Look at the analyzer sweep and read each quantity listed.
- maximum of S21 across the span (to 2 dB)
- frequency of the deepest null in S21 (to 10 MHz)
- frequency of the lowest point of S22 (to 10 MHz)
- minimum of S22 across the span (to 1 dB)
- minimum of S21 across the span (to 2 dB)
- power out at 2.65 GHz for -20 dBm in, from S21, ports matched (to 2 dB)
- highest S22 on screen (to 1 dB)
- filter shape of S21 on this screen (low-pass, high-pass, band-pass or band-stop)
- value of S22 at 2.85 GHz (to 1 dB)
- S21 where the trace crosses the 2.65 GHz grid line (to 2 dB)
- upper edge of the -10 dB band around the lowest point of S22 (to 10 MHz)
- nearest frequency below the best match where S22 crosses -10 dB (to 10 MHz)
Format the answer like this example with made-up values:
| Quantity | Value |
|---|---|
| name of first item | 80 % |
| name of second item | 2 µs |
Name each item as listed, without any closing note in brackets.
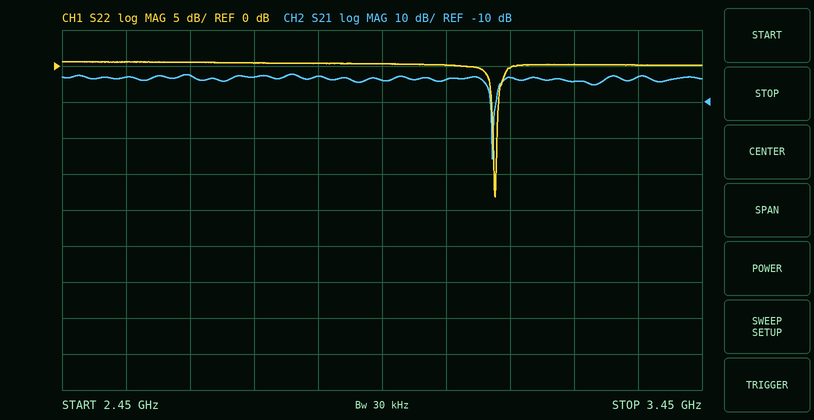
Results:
| Quantity | Value |
|---|---|
| maximum of S21 across the span | -2 dB |
| frequency of the deepest null in S21 | 3.12 GHz |
| frequency of the lowest point of S22 | 3.13 GHz |
| minimum of S22 across the span | -18 dB |
| minimum of S21 across the span | -26 dB |
| power out at 2.65 GHz for -20 dBm in, from S21, ports matched | -22 dBm |
| highest S22 on screen | 1 dB |
| filter shape of S21 on this screen | band-stop |
| value of S22 at 2.85 GHz | 0 dB |
| S21 where the trace crosses the 2.65 GHz grid line | -2 dB |
| upper edge of the -10 dB band around the lowest point of S22 | 3.13 GHz |
| nearest frequency below the best match where S22 crosses -10 dB | 3.12 GHz |
